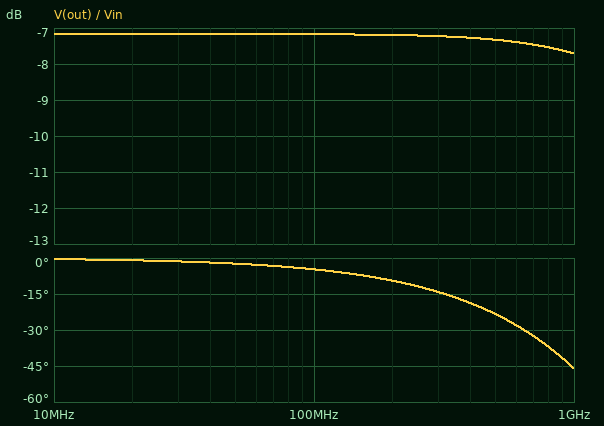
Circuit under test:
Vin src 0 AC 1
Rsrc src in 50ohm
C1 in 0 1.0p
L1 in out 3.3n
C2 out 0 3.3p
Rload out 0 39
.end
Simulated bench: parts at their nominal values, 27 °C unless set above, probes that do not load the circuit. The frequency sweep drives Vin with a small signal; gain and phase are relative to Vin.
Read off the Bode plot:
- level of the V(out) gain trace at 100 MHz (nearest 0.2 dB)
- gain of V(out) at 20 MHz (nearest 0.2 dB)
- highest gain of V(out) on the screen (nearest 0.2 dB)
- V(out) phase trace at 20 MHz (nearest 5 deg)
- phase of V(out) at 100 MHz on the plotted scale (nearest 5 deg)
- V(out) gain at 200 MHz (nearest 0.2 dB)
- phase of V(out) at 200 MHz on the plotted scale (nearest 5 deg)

-7.2 dB
-7.2 dB
-7.2 dB
0 deg
-5 deg
-7.2 dB
-10 deg
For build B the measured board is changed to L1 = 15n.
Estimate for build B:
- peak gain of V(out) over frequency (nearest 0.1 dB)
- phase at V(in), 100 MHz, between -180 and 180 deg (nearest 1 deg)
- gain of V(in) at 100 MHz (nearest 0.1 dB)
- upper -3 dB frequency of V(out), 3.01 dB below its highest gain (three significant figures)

-7.2 dB
4 deg
-7.1 dB
1.02 GHz
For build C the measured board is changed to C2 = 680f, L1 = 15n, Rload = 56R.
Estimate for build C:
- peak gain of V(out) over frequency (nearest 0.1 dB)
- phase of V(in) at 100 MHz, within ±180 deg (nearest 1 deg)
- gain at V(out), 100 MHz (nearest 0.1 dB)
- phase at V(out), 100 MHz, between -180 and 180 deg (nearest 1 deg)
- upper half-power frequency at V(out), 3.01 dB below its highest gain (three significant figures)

-5.5 dB
3 deg
-5.6 dB
-7 deg
1.35 GHz
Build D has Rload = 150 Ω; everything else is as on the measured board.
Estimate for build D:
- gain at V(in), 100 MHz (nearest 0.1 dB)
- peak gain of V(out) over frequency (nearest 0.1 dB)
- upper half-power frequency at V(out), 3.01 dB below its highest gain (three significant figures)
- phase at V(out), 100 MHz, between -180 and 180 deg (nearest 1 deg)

-2.6 dB
-2.5 dB
1.75 GHz
-6 deg
